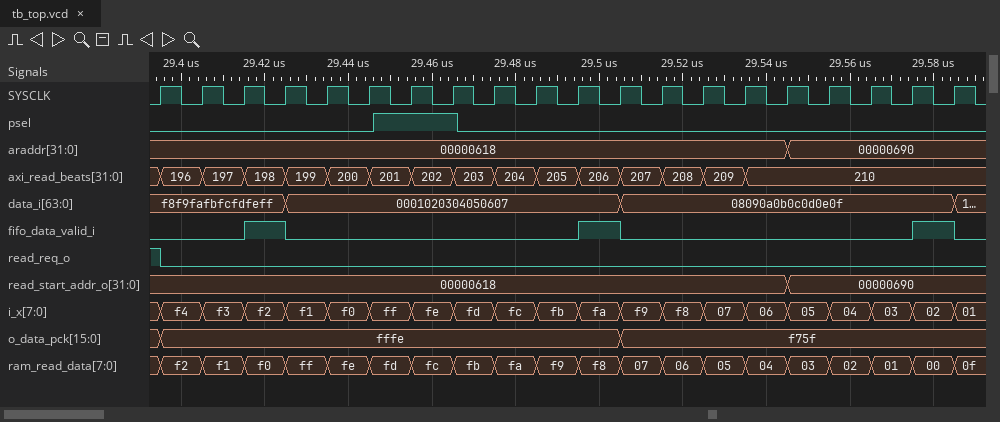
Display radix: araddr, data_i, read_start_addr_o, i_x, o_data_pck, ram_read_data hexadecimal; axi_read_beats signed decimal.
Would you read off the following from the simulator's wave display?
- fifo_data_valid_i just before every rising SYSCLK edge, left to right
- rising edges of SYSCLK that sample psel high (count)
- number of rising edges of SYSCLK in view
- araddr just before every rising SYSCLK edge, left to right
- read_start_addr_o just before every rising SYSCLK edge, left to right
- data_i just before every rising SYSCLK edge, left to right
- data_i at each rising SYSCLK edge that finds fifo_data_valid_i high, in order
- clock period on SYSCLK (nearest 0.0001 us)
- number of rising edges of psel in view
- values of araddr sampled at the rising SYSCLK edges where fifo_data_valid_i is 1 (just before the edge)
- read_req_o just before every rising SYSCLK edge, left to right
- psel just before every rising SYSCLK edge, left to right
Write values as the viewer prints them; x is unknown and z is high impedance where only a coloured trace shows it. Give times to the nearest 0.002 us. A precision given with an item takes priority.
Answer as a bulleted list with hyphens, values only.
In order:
- 0 0 0 1 0 0 0 0 0 0 0 1 0 0 0 0 0 0 0 1
- 2
- 20
- 00000618, 00000618, 00000618, 00000618, 00000618, 00000618, 00000618, 00000618, 00000618, 00000618, 00000618, 00000618, 00000618, 00000618, 00000618, 00000618, 00000690, 00000690, 00000690, 00000690
- 00000618, 00000618, 00000618, 00000618, 00000618, 00000618, 00000618, 00000618, 00000618, 00000618, 00000618, 00000618, 00000618, 00000618, 00000618, 00000618, 00000690, 00000690, 00000690, 00000690
- f8f9fafbfcfdfeff, f8f9fafbfcfdfeff, f8f9fafbfcfdfeff, f8f9fafbfcfdfeff, 0001020304050607, 0001020304050607, 0001020304050607, 0001020304050607, 0001020304050607, 0001020304050607, 0001020304050607, 0001020304050607, 08090a0b0c0d0e0f, 08090a0b0c0d0e0f, 08090a0b0c0d0e0f, 08090a0b0c0d0e0f, 08090a0b0c0d0e0f, 08090a0b0c0d0e0f, 08090a0b0c0d0e0f, 08090a0b0c0d0e0f
- f8f9fafbfcfdfeff, 0001020304050607, 08090a0b0c0d0e0f
- 0.01 us
- 1
- 00000618, 00000618, 00000690
- 1 0 0 0 0 0 0 0 0 0 0 0 0 0 0 0 0 0 0 0
- 0 0 0 0 0 0 1 1 0 0 0 0 0 0 0 0 0 0 0 0
